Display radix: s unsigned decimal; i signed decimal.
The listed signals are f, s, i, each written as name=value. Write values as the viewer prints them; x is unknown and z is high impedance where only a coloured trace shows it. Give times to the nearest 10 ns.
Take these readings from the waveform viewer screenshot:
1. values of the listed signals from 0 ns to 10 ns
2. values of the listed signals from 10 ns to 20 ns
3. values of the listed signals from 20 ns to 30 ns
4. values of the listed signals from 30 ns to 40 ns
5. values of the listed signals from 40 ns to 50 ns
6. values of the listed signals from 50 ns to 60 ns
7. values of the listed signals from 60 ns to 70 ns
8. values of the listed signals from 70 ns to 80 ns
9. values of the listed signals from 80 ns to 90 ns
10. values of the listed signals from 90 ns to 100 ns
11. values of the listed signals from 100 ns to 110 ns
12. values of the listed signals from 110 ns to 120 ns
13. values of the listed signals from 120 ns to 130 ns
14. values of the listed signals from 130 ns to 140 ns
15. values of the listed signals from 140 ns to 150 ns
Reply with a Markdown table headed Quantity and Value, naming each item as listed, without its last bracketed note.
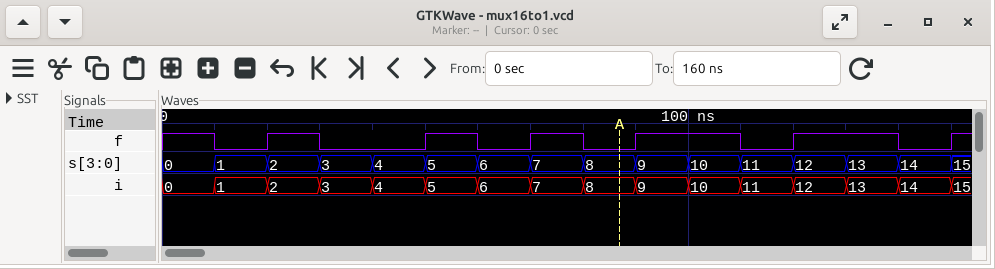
| Quantity | Value |
|---|---|
| values of the listed signals from 0 ns to 10 ns | f=1, s=0, i=0 |
| values of the listed signals from 10 ns to 20 ns | f=0, s=1, i=1 |
| values of the listed signals from 20 ns to 30 ns | f=1, s=2, i=2 |
| values of the listed signals from 30 ns to 40 ns | f=0, s=3, i=3 |
| values of the listed signals from 40 ns to 50 ns | f=0, s=4, i=4 |
| values of the listed signals from 50 ns to 60 ns | f=1, s=5, i=5 |
| values of the listed signals from 60 ns to 70 ns | f=0, s=6, i=6 |
| values of the listed signals from 70 ns to 80 ns | f=1, s=7, i=7 |
| values of the listed signals from 80 ns to 90 ns | f=0, s=8, i=8 |
| values of the listed signals from 90 ns to 100 ns | f=1, s=9, i=9 |
| values of the listed signals from 100 ns to 110 ns | f=1, s=10, i=10 |
| values of the listed signals from 110 ns to 120 ns | f=0, s=11, i=11 |
| values of the listed signals from 120 ns to 130 ns | f=1, s=12, i=12 |
| values of the listed signals from 130 ns to 140 ns | f=1, s=13, i=13 |
| values of the listed signals from 140 ns to 150 ns | f=0, s=14, i=14 |
